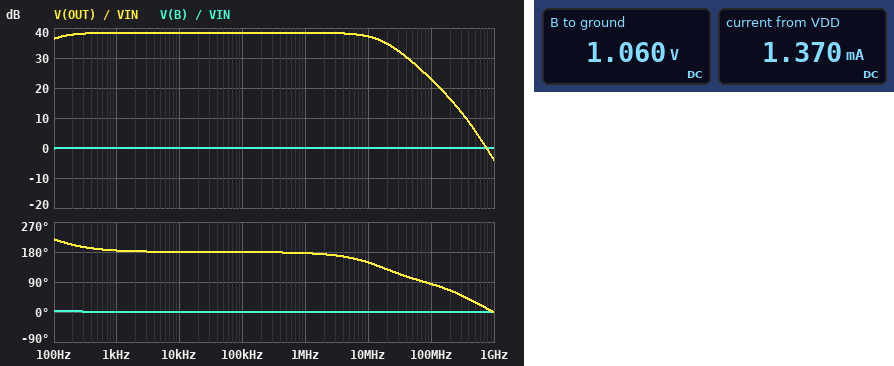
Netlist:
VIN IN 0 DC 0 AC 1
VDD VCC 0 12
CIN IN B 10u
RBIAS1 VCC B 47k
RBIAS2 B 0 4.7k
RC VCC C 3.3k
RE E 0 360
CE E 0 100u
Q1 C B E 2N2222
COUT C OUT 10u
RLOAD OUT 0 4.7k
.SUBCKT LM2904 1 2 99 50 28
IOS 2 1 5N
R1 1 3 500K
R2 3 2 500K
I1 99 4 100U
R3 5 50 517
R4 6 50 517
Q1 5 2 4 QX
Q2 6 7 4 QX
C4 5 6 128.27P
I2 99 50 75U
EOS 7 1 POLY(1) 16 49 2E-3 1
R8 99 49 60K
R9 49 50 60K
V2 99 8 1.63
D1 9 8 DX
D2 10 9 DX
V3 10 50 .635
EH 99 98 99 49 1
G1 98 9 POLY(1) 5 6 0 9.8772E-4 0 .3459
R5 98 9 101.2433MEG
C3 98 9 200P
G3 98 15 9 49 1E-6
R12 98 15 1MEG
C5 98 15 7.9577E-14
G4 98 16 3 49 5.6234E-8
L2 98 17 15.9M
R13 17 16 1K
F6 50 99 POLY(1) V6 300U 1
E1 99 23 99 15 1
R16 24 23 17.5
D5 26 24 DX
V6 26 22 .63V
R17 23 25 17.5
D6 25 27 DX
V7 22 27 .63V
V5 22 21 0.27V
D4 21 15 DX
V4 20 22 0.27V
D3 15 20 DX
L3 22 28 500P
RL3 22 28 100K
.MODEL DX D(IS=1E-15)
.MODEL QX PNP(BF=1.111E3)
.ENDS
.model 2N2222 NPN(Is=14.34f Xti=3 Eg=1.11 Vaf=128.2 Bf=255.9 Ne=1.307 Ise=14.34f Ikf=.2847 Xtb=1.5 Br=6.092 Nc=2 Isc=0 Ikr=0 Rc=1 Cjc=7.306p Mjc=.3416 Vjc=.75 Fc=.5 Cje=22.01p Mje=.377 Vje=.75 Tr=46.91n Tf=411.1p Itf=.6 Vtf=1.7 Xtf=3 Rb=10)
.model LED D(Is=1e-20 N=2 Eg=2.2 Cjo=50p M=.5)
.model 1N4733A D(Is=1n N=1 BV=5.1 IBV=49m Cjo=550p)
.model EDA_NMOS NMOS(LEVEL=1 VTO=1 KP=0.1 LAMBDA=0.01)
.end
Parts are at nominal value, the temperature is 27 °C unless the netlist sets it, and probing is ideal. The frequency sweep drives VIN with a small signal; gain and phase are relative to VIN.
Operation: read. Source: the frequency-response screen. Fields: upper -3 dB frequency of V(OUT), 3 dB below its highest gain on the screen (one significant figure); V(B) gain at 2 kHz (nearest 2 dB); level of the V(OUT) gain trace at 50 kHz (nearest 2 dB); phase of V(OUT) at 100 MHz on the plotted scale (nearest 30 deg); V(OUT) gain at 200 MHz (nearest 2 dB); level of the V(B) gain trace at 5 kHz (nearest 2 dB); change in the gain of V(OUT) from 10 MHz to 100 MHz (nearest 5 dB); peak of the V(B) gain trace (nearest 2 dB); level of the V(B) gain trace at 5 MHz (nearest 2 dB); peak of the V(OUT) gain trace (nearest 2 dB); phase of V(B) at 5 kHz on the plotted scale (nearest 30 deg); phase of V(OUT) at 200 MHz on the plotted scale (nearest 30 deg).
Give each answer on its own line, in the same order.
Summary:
20 MHz
0 dB
38 dB
90 deg
16 dB
0 dB
-15 dB
0 dB
0 dB
38 dB
0 deg
60 deg
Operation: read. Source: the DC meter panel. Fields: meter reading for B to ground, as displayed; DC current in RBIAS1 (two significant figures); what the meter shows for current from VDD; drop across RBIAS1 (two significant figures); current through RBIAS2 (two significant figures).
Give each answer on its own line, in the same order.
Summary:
1.060 V
230 µA
1.370 mA
11 V
230 µA
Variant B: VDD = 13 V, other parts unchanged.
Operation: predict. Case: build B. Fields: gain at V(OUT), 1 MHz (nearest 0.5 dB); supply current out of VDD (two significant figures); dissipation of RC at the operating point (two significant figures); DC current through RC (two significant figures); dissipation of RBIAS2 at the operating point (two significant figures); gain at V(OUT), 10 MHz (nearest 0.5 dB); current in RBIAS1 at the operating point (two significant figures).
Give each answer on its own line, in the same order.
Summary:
40.0 dB
1.6 mA
6.1 mW
1.4 mA
280 µW
38.5 dB
250 µA
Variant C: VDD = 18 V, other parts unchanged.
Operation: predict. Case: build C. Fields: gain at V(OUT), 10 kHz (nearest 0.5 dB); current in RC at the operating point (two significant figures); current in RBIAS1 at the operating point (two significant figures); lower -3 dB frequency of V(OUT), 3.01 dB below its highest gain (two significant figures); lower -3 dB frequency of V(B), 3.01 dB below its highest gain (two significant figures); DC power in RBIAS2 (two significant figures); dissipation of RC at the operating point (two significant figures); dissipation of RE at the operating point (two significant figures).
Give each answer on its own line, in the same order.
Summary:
45.0 dB
2.5 mA
350 µA
160 Hz
4.2 Hz
530 µW
21 mW
2.3 mW
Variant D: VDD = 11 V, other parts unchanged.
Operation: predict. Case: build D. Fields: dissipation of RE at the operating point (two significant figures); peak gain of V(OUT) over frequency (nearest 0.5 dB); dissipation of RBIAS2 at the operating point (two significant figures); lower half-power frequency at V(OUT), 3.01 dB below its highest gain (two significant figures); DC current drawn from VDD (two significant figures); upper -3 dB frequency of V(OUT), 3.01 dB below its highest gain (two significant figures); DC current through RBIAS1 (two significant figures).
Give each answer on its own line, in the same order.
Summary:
310 µW
36.5 dB
200 µW
63 Hz
1.1 mA
18 MHz
210 µA
